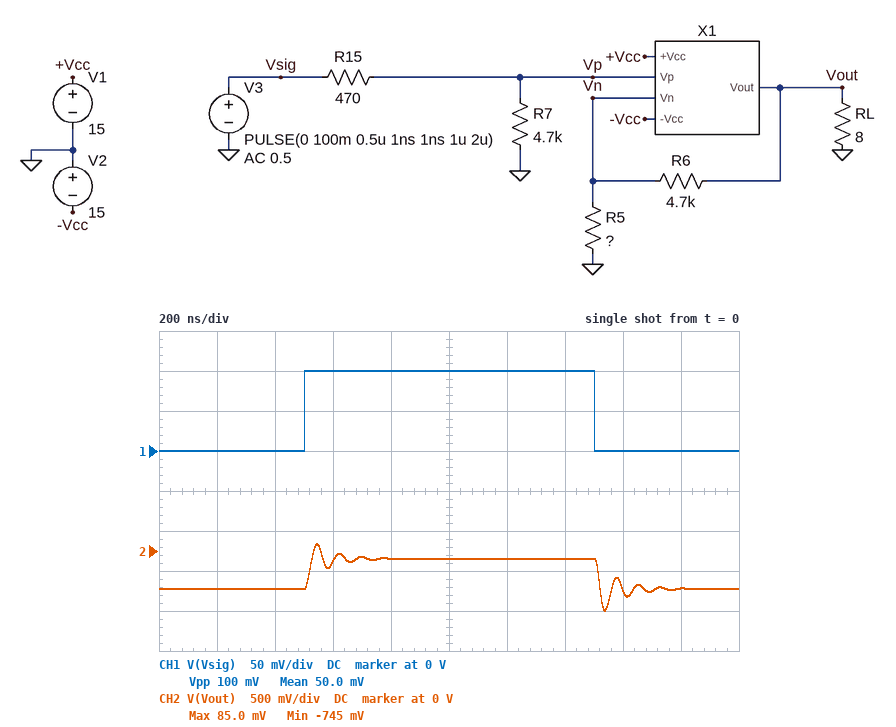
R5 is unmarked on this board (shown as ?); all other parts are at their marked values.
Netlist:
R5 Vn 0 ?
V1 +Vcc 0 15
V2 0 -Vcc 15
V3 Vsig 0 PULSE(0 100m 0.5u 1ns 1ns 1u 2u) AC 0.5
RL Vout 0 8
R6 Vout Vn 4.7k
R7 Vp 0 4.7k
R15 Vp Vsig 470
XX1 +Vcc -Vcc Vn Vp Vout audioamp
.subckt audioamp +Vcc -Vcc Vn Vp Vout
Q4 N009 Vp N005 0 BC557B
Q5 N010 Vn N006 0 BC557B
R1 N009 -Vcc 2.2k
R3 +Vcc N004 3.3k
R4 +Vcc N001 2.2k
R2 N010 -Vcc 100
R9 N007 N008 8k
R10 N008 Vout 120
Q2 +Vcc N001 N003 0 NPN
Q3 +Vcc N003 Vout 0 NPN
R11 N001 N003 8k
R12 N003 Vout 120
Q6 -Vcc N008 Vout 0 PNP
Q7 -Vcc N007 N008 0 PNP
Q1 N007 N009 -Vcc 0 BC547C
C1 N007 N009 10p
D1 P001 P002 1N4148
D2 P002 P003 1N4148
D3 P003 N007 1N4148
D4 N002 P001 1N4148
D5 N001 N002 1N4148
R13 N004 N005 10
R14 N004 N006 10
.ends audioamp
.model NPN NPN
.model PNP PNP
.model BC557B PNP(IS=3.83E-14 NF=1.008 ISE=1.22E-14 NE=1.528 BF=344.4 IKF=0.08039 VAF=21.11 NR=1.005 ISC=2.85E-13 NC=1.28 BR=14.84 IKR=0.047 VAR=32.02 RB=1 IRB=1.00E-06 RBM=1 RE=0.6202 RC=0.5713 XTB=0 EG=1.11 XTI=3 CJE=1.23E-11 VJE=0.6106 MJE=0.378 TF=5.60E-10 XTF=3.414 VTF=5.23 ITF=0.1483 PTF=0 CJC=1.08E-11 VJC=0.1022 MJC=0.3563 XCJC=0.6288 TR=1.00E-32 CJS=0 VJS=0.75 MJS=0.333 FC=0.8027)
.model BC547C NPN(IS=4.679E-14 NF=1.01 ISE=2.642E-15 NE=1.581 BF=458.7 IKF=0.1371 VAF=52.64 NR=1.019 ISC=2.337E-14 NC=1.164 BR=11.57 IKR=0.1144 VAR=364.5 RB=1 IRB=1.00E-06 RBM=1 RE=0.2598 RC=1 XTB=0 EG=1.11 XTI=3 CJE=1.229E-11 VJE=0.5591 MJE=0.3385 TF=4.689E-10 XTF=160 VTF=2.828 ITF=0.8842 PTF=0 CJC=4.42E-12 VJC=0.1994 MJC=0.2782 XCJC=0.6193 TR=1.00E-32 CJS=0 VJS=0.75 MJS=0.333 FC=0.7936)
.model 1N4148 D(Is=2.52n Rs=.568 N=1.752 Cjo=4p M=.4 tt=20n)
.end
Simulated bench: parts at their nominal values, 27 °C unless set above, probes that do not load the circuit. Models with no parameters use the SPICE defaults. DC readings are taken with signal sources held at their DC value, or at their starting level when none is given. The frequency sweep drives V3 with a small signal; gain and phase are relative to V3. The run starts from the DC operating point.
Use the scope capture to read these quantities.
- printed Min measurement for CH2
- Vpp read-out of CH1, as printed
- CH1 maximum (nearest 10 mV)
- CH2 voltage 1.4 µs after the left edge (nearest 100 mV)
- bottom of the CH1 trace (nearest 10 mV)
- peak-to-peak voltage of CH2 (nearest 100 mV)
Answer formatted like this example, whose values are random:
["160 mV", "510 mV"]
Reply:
["-745 mV", "100 mV", "100 mV", "-100 mV", "0 V", "800 mV"]
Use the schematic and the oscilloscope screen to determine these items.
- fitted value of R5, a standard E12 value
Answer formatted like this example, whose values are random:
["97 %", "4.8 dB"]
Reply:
["1.5 kΩ"]
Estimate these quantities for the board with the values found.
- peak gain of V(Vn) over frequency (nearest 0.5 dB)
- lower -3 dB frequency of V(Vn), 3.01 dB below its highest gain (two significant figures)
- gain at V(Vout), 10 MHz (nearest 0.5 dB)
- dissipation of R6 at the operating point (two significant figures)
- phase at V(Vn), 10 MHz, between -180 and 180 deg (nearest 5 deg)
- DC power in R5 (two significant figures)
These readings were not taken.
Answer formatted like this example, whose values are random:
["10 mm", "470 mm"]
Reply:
["5.5 dB", "9.6 MHz", "17.5 dB", "29 µW", "-40 deg", "7.6 µW"]
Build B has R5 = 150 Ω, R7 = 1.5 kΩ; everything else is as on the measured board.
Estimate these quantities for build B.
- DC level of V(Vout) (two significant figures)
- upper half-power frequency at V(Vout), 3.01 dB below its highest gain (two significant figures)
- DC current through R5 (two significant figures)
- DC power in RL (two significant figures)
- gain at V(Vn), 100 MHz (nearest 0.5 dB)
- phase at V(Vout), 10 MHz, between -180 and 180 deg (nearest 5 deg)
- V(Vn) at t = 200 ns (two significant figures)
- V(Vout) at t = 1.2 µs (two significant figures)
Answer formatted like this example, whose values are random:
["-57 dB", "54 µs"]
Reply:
["-3.5 V", "5.0 MHz", "710 µA", "1.5 W", "-17.5 dB", "-115 deg", "-110 mV", "-1.0 V"]
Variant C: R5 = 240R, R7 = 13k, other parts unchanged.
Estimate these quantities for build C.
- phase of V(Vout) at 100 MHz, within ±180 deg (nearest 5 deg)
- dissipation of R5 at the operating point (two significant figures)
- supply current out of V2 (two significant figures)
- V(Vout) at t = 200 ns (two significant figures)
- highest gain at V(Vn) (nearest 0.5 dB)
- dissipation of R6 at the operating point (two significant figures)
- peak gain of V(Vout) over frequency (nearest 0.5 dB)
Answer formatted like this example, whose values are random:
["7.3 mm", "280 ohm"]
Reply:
["150 deg", "47 µW", "300 mA", "-2.2 V", "-0.5 dB", "950 µW", "26.0 dB"]
